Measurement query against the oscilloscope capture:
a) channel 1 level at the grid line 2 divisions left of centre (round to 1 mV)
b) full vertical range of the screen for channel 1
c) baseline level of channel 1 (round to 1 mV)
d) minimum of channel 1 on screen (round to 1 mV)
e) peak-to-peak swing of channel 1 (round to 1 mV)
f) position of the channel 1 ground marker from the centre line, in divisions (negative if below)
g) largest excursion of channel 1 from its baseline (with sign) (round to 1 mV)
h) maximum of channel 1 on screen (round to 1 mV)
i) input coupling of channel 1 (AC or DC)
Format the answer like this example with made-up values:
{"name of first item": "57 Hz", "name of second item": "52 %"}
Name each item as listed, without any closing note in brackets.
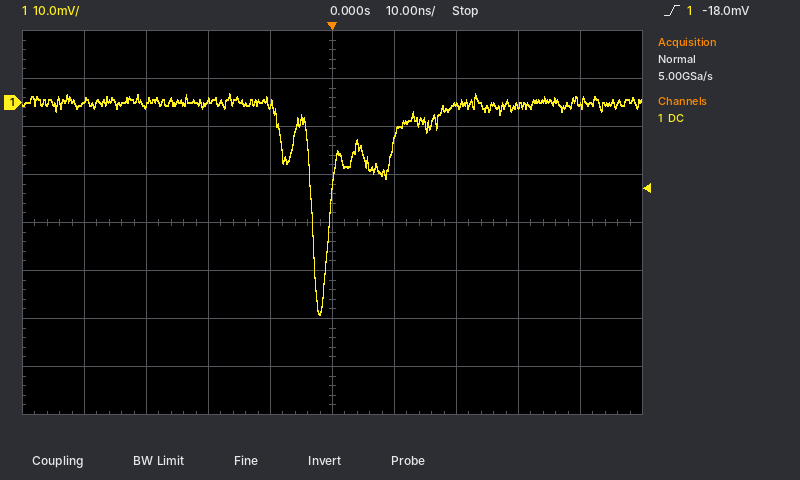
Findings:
{"channel 1 level at the grid line 2 divisions left of centre": "0 mV", "full vertical range of the screen for channel 1": "80 mV", "baseline level of channel 1": "0 mV", "minimum of channel 1 on screen": "-44 mV", "peak-to-peak swing of channel 1": "46 mV", "position of the channel 1 ground marker from the centre line, in divisions": "+2.5 div", "largest excursion of channel 1 from its baseline (with sign)": "-44 mV", "maximum of channel 1 on screen": "2 mV", "input coupling of channel 1": "DC"}
